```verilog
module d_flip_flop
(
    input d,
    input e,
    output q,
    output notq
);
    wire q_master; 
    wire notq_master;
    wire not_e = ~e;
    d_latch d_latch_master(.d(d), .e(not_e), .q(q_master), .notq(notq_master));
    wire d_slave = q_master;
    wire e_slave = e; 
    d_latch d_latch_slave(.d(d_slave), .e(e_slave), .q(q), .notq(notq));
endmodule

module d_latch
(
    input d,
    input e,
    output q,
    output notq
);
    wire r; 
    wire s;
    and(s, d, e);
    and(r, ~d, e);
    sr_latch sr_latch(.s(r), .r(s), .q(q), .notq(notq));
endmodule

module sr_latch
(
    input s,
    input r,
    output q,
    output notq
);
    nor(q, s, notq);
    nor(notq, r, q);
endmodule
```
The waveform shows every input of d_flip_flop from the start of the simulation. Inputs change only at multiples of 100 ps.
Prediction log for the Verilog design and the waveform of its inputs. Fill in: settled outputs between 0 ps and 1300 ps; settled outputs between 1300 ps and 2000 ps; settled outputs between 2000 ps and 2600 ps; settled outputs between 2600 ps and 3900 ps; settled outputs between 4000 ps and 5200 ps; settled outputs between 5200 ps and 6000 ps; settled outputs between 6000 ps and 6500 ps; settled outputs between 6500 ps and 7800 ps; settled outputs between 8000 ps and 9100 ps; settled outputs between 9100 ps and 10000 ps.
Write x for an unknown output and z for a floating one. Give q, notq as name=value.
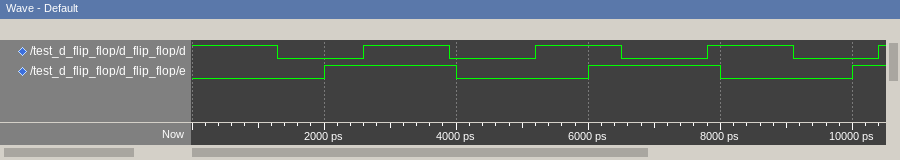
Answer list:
q=x, notq=x
q=x, notq=x
q=0, notq=1
q=0, notq=1
q=0, notq=1
q=0, notq=1
q=1, notq=0
q=1, notq=0
q=1, notq=0
q=1, notq=0
